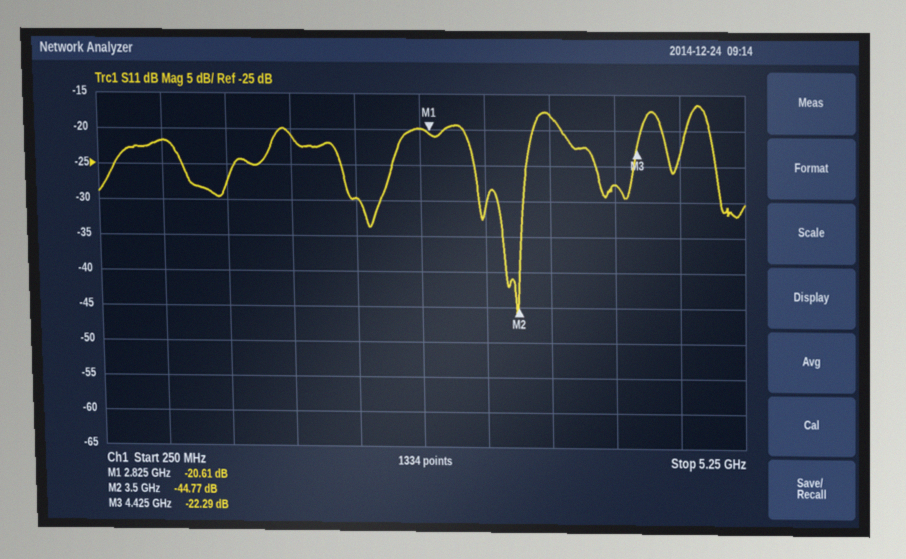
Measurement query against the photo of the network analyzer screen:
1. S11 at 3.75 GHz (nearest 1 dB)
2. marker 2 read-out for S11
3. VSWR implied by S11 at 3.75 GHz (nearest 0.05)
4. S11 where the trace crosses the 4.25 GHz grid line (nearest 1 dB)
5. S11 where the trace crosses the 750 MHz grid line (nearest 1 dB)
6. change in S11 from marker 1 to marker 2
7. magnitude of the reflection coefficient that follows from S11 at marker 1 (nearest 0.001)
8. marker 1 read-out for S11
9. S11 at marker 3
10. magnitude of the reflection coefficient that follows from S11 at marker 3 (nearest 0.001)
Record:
-18 dB
-44.77 dB
1.30
-28 dB
-22 dB
-24.16 dB
0.093
-20.61 dB
-22.29 dB
0.077
